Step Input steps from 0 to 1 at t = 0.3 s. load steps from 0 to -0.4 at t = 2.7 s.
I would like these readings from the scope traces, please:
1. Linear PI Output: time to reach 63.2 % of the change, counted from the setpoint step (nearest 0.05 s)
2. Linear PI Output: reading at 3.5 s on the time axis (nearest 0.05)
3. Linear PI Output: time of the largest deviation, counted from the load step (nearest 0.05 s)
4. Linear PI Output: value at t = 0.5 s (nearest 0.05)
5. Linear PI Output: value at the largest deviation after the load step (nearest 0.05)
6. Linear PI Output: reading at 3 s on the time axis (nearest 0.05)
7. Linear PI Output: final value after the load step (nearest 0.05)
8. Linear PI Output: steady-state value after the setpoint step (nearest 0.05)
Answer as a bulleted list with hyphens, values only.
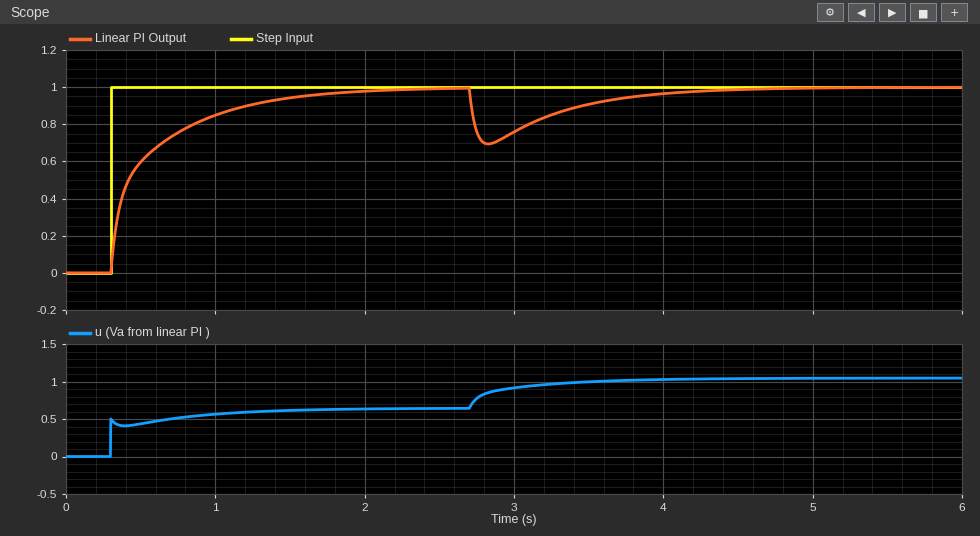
- 0.25 s
- 0.90
- 0.15 s
- 0.60
- 0.70
- 0.75
- 1.00
- 1.00
